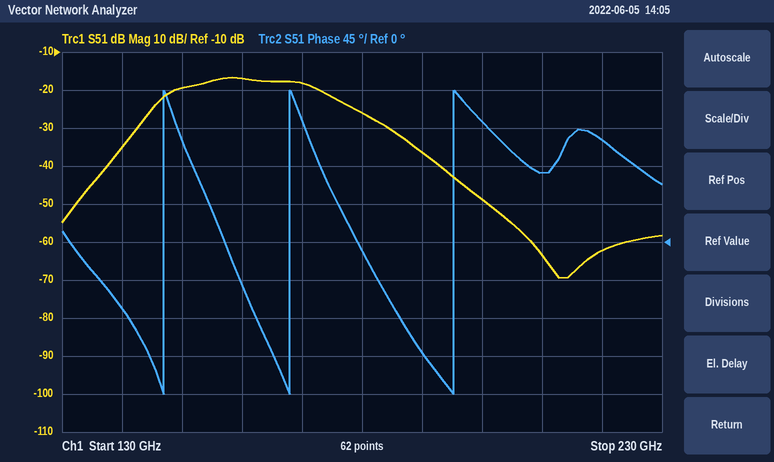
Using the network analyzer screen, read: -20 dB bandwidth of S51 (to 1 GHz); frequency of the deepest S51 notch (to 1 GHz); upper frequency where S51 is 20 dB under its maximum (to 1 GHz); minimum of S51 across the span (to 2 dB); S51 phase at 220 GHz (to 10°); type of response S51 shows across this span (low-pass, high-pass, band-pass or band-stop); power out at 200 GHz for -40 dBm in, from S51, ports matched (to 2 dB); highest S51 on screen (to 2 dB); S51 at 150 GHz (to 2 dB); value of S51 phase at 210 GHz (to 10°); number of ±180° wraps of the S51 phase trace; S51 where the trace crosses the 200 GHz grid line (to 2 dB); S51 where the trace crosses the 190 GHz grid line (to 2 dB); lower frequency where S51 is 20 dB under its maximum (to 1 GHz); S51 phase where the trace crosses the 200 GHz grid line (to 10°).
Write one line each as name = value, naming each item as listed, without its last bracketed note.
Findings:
-20 dB bandwidth of S51 = 51 GHz
frequency of the deepest S51 notch = 213 GHz
upper frequency where S51 is 20 dB under its maximum = 190 GHz
minimum of S51 across the span = -70 dB
S51 phase at 220 GHz = 120°
type of response S51 shows across this span = band-pass
power out at 200 GHz for -40 dBm in, from S51, ports matched = -88 dBm
highest S51 on screen = -16 dB
S51 at 150 GHz = -20 dB
value of S51 phase at 210 GHz = 80°
number of ±180° wraps of the S51 phase trace = 3
S51 where the trace crosses the 200 GHz grid line = -48 dB
S51 where the trace crosses the 190 GHz grid line = -36 dB
lower frequency where S51 is 20 dB under its maximum = 139 GHz
S51 phase where the trace crosses the 200 GHz grid line = 140°
